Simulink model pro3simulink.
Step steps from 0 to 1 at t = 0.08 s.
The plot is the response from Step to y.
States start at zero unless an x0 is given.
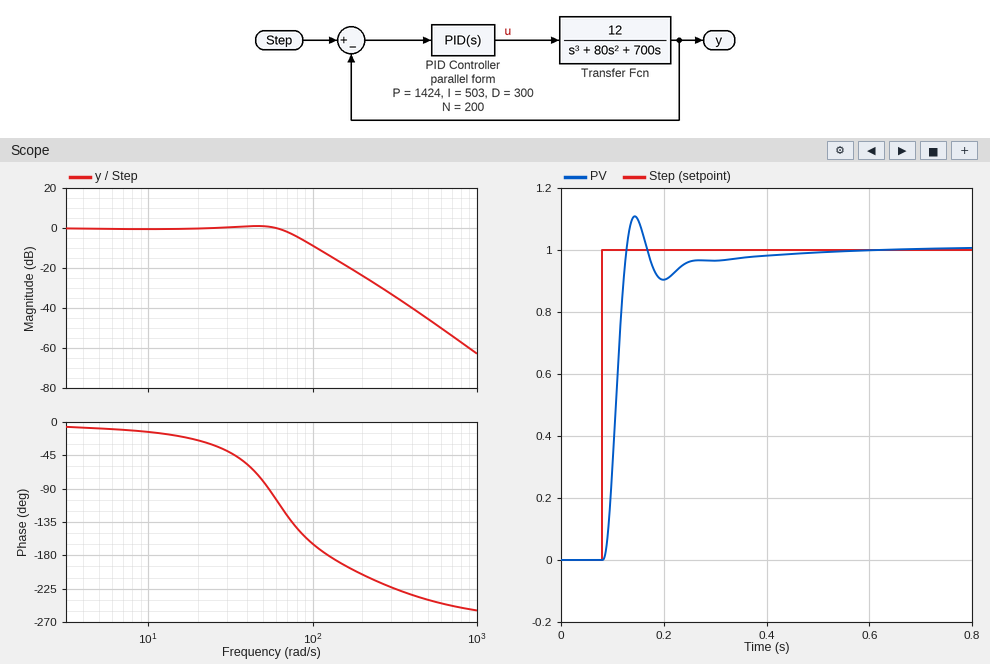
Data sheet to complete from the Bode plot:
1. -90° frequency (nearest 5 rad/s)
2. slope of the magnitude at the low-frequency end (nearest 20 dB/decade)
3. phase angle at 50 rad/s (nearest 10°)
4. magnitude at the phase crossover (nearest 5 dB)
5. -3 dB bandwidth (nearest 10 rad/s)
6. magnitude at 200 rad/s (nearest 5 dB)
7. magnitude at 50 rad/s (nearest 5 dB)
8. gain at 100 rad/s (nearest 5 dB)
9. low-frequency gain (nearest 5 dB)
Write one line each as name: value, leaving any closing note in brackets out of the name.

-90° frequency: 55 rad/s
slope of the magnitude at the low-frequency end: 0 dB/decade
phase angle at 50 rad/s: -80°
magnitude at the phase crossover: -15 dB
-3 dB bandwidth: 80 rad/s
magnitude at 200 rad/s: -25 dB
magnitude at 50 rad/s: 0 dB
gain at 100 rad/s: -10 dB
low-frequency gain: 0 dB
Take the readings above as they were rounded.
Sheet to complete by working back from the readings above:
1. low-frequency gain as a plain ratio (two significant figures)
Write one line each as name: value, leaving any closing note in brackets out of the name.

low-frequency gain as a plain ratio: 1.0
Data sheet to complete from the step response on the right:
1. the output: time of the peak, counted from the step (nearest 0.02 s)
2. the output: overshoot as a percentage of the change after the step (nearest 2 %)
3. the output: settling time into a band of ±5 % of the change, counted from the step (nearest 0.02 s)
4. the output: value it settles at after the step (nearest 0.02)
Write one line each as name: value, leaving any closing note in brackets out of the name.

the output: time of the peak, counted from the step: 0.06 s
the output: overshoot as a percentage of the change after the step: 10 %
the output: settling time into a band of ±5 % of the change, counted from the step: 0.16 s
the output: value it settles at after the step: 1.00
